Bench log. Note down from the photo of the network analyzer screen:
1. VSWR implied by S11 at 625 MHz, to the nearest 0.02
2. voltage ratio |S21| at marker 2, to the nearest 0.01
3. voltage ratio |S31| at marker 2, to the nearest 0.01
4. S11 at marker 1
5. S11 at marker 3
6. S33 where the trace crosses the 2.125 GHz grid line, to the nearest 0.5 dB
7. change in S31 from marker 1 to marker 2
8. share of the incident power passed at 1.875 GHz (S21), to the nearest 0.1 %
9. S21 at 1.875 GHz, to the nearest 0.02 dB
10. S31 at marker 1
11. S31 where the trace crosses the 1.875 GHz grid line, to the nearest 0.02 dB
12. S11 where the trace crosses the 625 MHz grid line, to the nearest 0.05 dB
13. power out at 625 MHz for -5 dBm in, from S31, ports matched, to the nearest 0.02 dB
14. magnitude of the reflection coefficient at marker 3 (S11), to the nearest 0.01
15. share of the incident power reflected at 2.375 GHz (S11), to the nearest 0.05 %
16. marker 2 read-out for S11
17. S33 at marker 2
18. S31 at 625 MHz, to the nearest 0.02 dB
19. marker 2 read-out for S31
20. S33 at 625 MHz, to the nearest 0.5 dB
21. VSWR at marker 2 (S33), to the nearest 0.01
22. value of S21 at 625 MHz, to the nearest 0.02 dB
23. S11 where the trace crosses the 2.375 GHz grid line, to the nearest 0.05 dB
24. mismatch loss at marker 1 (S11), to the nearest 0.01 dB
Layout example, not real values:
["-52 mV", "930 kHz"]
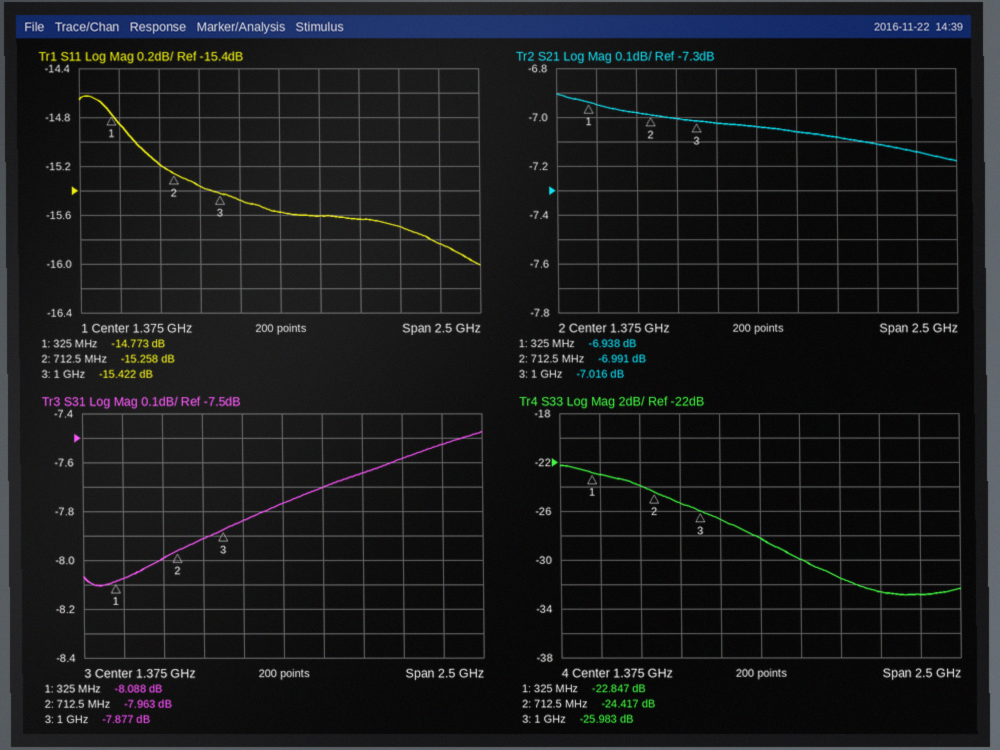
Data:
["1.42", "0.45", "0.40", "-14.773 dB", "-15.422 dB", "-32.5 dB", "0.125 dB", "19.6 %", "-7.08 dB", "-8.088 dB", "-7.64 dB", "-15.20 dB", "-13.00 dBm", "0.17", "2.60 %", "-15.258 dB", "-24.417 dB", "-8.00 dB", "-7.963 dB", "-24.0 dB", "1.13", "-6.98 dB", "-15.85 dB", "0.15 dB"]
